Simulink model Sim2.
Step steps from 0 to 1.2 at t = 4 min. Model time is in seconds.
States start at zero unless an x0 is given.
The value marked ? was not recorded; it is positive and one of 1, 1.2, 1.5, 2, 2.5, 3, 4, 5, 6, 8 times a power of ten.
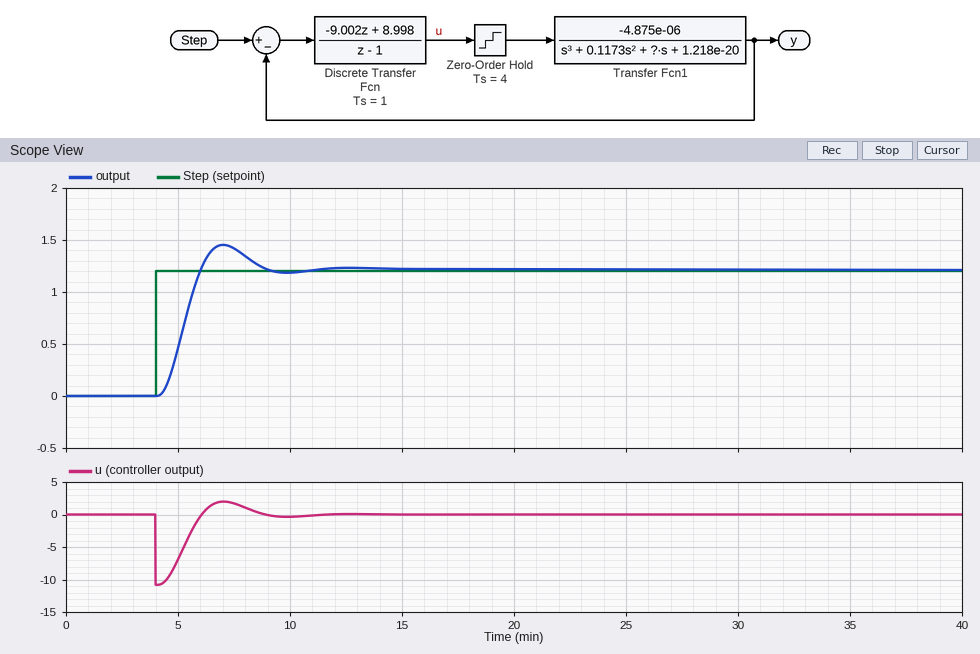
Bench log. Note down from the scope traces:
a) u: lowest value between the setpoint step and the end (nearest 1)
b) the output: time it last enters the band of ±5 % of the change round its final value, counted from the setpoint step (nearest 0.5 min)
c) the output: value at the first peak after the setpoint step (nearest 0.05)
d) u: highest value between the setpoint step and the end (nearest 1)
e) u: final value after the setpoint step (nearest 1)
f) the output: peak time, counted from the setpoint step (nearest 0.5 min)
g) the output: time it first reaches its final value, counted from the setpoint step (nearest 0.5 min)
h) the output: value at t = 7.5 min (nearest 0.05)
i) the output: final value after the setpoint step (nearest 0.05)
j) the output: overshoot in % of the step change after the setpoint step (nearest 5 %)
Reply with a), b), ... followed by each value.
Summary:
a) -11
b) 4.5 min
c) 1.45
d) 2
e) 0
f) 3.0 min
g) 2.0 min
h) 1.40
i) 1.20
j) 20 %
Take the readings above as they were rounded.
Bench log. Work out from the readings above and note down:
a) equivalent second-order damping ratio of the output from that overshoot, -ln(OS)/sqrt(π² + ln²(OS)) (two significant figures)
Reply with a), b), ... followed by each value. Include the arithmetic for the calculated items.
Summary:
a) ln(0.2) = -1.609; 1.609 / sqrt(9.870 + 2.590) = 0.46
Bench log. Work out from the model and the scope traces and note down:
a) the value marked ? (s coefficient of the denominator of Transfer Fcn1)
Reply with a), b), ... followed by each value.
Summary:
a) 0.0025
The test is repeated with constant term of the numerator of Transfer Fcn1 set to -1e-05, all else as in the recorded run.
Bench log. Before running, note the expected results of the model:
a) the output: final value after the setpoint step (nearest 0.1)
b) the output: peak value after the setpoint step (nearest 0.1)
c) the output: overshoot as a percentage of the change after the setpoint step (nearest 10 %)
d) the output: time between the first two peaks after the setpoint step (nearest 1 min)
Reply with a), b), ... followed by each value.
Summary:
a) 1.2
b) 1.8
c) 50 %
d) 4 min
